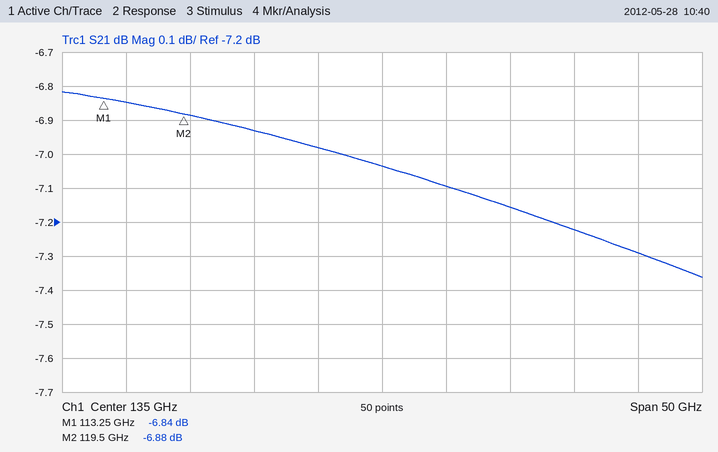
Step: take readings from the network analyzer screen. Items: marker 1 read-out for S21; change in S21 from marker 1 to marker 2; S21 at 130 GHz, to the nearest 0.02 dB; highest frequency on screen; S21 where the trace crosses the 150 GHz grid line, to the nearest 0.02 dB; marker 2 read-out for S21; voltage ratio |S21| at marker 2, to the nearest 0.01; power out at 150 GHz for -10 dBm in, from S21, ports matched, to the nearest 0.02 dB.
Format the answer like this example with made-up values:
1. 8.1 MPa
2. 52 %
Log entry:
1. -6.84 dB
2. -0.04 dB
3. -6.98 dB
4. 160 GHz
5. -7.22 dB
6. -6.88 dB
7. 0.45
8. -17.22 dBm
